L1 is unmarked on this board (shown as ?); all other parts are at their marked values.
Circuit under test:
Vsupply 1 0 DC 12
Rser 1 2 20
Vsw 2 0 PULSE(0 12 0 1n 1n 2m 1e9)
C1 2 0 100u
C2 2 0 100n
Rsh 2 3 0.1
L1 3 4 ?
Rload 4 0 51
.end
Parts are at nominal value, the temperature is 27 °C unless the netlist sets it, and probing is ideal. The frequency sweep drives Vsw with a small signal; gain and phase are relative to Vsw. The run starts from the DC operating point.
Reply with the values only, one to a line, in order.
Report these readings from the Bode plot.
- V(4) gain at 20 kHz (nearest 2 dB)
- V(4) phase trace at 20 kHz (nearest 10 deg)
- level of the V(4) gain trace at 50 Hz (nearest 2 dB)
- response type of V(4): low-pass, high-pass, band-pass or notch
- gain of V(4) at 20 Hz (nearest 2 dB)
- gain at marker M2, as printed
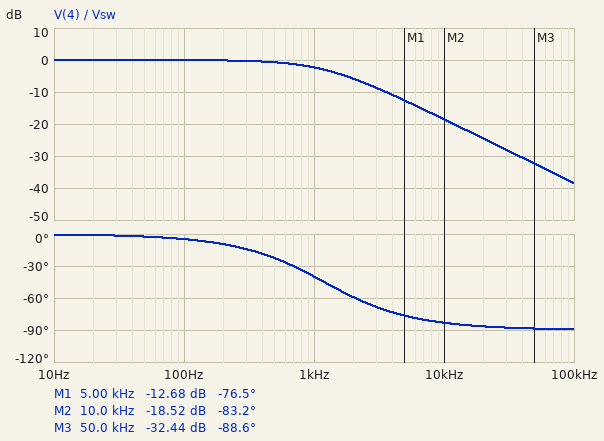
-24 dB
-90 deg
0 dB
low-pass
0 dB
-18.52 dB
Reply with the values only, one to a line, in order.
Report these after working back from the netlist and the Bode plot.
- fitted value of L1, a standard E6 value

6.8 mH
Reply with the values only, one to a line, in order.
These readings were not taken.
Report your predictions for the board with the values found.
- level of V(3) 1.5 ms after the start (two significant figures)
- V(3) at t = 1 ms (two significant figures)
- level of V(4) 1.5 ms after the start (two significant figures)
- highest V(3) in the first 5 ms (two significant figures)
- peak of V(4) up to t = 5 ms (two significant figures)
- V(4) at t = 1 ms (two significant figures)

12 V
12 V
12 V
12 V
12 V
12 V
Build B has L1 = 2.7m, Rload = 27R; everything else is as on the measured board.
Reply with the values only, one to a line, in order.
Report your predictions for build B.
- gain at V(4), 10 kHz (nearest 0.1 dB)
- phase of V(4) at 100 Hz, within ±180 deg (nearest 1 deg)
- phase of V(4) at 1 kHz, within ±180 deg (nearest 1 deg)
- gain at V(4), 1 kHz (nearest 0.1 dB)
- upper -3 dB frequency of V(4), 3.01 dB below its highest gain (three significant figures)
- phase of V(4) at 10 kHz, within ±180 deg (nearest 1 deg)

-16.1 dB
-4 deg
-32 deg
-1.5 dB
1.60 kHz
-81 deg
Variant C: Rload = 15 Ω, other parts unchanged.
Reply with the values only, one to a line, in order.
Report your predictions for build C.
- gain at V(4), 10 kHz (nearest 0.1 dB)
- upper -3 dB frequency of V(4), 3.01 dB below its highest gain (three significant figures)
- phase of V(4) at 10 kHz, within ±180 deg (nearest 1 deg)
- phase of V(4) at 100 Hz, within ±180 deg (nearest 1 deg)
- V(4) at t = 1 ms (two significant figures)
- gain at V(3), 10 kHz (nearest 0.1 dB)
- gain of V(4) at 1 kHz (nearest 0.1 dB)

-29.1 dB
353 Hz
-88 deg
-16 deg
11 V
0 dB
-9.6 dB
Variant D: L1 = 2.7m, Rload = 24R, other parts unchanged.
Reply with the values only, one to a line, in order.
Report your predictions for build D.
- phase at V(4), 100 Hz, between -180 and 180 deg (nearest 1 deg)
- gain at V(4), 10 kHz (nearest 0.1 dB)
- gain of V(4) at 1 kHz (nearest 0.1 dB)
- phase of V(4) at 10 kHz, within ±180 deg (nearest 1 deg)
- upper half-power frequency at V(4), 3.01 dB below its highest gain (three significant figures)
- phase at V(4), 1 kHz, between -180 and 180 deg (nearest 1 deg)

-4 deg
-17.1 dB
-1.8 dB
-82 deg
1.42 kHz
-35 deg
